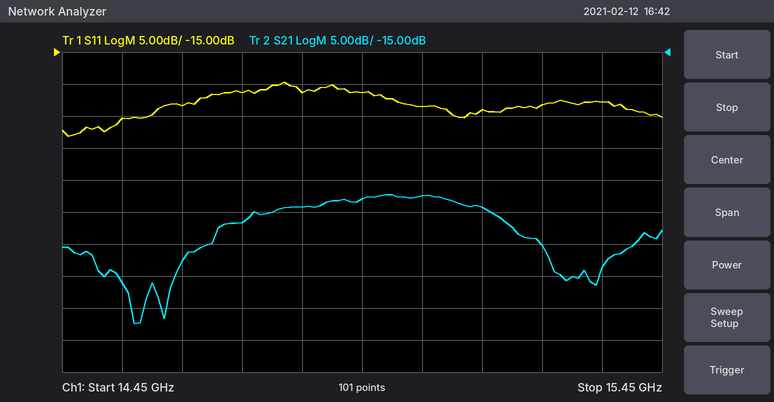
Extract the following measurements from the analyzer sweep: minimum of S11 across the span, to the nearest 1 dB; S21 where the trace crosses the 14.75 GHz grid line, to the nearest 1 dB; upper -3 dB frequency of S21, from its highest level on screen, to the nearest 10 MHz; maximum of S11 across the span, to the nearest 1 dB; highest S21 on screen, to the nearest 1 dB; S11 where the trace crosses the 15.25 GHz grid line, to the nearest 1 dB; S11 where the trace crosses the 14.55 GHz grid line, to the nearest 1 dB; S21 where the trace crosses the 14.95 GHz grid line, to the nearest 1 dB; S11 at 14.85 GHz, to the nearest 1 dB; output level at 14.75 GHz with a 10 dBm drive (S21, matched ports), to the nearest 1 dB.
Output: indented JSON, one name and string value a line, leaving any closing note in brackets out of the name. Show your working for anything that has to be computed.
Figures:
{
  "minimum of S11 across the span, to the nearest 1 dB": "-28 dB",
  "S21 where the trace crosses the 14.75 GHz grid line, to the nearest 1 dB": "-42 dB",
  "upper -3 dB frequency of S21, from its highest level on screen, to the nearest 10 MHz": "15.17 GHz",
  "maximum of S11 across the span, to the nearest 1 dB": "-20 dB",
  "highest S21 on screen, to the nearest 1 dB": "-37 dB",
  "S11 where the trace crosses the 15.25 GHz grid line, to the nearest 1 dB": "-23 dB",
  "S11 where the trace crosses the 14.55 GHz grid line, to the nearest 1 dB": "-25 dB",
  "S21 where the trace crosses the 14.95 GHz grid line, to the nearest 1 dB": "-38 dB",
  "S11 at 14.85 GHz, to the nearest 1 dB": "-21 dB",
  "output level at 14.75 GHz with a 10 dBm drive (S21, matched ports), to the nearest 1 dB": "10 dBm + (-42 dB) = -32 dBm"
}
